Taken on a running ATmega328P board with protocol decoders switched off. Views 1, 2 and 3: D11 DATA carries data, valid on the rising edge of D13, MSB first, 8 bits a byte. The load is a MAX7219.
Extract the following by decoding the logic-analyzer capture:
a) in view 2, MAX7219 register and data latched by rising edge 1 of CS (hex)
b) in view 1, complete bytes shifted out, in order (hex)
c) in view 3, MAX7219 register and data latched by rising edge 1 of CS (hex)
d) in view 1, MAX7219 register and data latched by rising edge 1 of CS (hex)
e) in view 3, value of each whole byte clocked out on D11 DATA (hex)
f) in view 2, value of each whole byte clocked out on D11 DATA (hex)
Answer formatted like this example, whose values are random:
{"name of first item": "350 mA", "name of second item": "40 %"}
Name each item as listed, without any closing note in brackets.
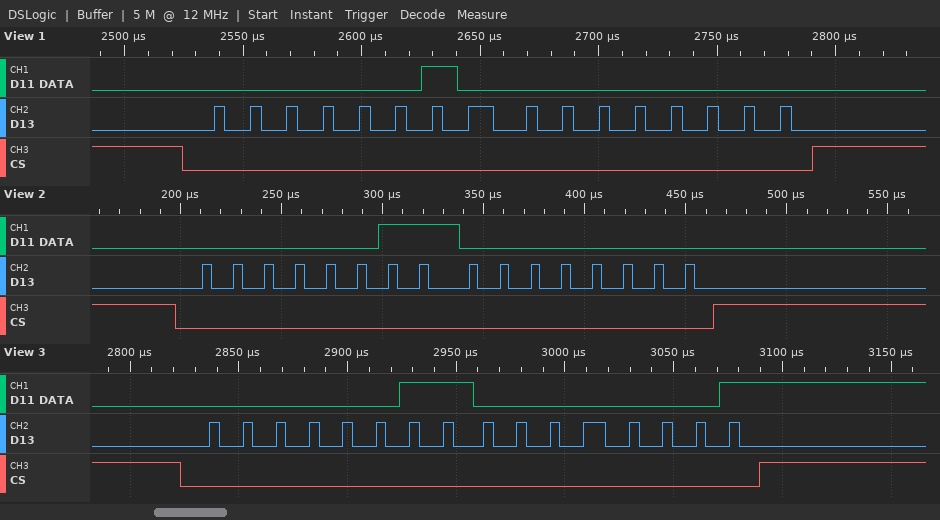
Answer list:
{"in view 2, MAX7219 register and data latched by rising edge 1 of CS": "register 0x3, data 0x00", "in view 1, complete bytes shifted out, in order": "02 00", "in view 3, MAX7219 register and data latched by rising edge 1 of CS": "register 0x3, data 0x01", "in view 1, MAX7219 register and data latched by rising edge 1 of CS": "register 0x2, data 0x00", "in view 3, value of each whole byte clocked out on D11 DATA": "03 01", "in view 2, value of each whole byte clocked out on D11 DATA": "0x03 0x00"}
